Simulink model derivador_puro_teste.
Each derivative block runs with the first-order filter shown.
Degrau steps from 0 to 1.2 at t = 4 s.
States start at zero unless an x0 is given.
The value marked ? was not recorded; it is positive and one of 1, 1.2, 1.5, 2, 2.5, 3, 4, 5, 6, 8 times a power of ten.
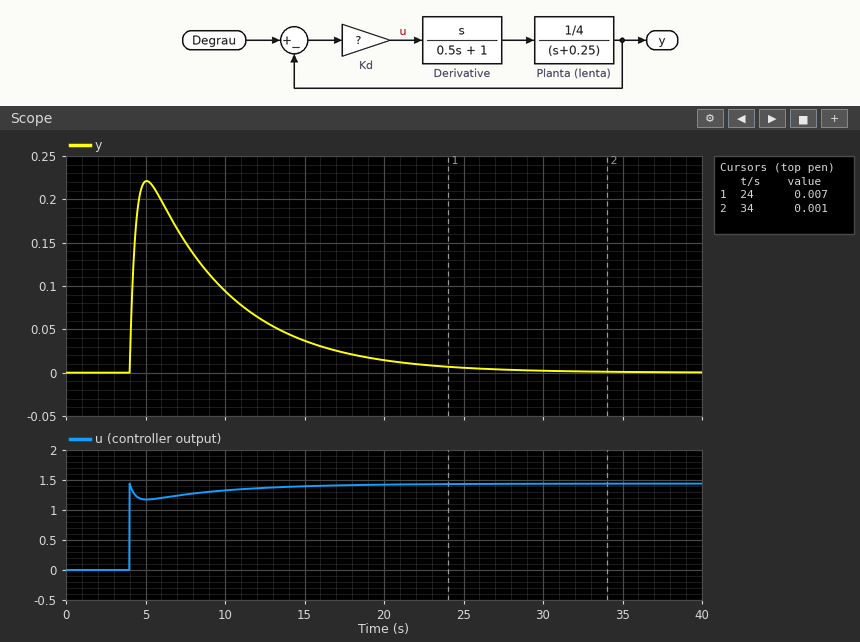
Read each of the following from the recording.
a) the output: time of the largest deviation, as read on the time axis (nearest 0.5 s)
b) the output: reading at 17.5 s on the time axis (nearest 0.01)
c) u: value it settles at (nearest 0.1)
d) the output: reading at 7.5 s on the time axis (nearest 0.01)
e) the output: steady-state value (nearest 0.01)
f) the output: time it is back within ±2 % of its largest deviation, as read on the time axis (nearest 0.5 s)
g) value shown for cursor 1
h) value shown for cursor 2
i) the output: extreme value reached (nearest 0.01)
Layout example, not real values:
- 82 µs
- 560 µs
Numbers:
- 5.0 s
- 0.02
- 1.4
- 0.15
- 0.00
- 26.5 s
- 0.007
- 0.001
- 0.22
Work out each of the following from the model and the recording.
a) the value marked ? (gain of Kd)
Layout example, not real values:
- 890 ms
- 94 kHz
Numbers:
- 1.2
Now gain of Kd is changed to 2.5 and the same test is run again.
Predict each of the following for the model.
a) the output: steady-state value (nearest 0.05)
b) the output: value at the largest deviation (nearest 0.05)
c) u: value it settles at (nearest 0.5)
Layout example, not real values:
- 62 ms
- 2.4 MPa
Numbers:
- 0.00
- 0.40
- 3.0
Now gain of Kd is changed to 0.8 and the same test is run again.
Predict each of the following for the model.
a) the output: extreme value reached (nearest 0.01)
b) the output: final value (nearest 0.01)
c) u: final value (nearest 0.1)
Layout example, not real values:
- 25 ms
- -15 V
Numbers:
- 0.16
- 0.00
- 1.0
